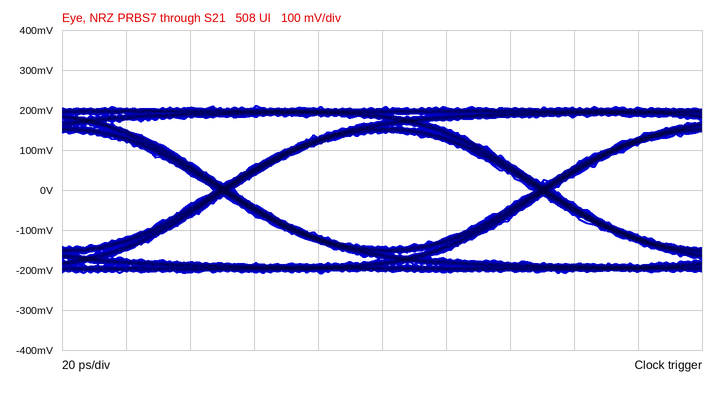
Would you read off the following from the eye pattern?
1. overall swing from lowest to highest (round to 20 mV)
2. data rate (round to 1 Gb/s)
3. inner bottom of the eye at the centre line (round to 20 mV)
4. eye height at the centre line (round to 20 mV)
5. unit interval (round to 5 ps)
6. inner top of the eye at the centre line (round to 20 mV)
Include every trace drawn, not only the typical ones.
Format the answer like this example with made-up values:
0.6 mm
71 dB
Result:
420 mV
10 Gb/s
-140 mV
280 mV
100 ps
140 mV
